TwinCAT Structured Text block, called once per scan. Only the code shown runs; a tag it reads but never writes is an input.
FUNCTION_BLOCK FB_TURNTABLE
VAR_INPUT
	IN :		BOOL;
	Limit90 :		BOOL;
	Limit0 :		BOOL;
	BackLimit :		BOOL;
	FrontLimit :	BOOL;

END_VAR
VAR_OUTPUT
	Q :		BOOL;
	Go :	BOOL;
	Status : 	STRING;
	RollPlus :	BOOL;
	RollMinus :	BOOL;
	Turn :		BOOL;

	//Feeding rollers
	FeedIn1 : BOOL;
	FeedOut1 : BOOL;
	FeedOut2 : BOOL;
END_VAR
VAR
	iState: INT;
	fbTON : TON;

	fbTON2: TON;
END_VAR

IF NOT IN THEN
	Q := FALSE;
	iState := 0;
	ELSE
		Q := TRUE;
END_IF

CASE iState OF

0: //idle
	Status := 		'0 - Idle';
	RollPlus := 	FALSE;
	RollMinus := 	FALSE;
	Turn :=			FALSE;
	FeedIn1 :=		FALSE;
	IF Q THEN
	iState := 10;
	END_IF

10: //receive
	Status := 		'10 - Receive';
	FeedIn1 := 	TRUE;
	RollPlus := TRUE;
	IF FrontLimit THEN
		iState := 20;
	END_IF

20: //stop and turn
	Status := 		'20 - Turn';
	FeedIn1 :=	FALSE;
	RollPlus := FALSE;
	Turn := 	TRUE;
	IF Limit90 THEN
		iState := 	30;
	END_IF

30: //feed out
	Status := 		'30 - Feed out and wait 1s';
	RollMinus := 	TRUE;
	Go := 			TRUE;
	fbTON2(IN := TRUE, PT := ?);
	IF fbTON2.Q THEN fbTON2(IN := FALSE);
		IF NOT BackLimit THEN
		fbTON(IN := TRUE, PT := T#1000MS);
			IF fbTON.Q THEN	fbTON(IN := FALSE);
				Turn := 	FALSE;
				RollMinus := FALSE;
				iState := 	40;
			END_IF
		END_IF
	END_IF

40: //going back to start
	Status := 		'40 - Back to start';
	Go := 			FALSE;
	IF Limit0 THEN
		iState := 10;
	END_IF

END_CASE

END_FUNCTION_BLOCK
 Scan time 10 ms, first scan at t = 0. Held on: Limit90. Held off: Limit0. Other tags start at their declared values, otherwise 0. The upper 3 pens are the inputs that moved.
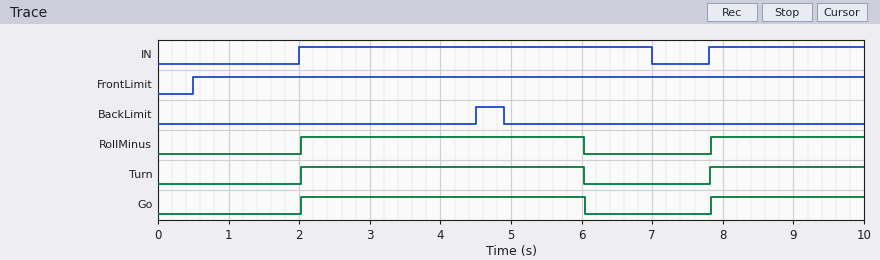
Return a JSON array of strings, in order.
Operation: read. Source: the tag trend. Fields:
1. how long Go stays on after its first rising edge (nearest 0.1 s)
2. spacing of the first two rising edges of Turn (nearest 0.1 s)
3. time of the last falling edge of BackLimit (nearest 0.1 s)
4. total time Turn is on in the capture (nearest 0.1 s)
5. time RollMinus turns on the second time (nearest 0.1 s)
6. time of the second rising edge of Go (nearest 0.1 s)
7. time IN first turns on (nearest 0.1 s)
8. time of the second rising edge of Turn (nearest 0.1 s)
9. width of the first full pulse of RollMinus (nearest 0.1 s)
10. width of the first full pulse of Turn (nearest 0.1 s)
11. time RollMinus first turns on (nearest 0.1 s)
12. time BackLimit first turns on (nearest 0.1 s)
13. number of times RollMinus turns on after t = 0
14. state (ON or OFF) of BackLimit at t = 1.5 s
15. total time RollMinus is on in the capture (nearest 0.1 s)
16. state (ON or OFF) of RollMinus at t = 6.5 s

["4.0 s", "5.8 s", "4.9 s", "6.2 s", "7.8 s", "7.8 s", "2.0 s", "7.8 s", "4.0 s", "4.0 s", "2.0 s", "4.5 s", "2", "OFF", "6.2 s", "OFF"]
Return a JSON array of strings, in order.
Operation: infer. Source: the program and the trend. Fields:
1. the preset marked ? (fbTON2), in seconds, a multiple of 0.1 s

["2.0 s"]
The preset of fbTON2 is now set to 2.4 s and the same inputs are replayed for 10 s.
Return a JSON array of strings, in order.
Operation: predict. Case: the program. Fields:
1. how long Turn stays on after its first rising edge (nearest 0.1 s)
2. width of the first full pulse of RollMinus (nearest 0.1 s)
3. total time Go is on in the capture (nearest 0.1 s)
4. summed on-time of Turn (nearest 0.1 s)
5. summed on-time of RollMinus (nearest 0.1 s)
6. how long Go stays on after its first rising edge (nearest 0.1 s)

["4.8 s", "4.8 s", "7.0 s", "7.0 s", "7.0 s", "4.8 s"]
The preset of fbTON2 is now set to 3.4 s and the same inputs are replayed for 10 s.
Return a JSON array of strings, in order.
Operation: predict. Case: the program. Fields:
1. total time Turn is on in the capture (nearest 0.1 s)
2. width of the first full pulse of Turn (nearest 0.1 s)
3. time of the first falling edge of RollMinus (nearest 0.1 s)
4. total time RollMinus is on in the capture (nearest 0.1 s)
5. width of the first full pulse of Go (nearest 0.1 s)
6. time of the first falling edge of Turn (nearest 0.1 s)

["6.0 s", "5.0 s", "7.0 s", "6.0 s", "6.8 s", "7.0 s"]
